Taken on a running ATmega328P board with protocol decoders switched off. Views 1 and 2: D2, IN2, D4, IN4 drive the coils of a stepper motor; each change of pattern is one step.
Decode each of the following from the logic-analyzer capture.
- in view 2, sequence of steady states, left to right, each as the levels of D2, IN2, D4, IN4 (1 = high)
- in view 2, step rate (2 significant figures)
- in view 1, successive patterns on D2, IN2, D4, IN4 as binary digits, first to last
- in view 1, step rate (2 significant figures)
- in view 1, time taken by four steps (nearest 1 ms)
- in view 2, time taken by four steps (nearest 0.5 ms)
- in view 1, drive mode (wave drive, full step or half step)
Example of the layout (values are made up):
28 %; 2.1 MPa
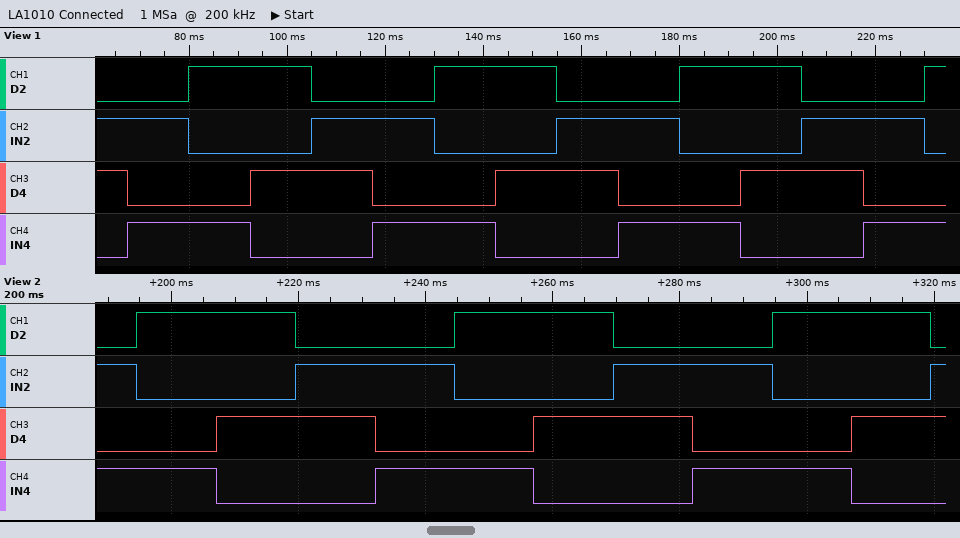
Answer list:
0101 1001 1010 0110 0101 1001 1010 0110 0101 1001 1010 0110; 80 steps/s; 0110 0101 1001 1010 0110 0101 1001 1010 0110 0101 1001 1010 0110 0101 1001; 80 steps/s; 50 ms; 50.0 ms; full step
